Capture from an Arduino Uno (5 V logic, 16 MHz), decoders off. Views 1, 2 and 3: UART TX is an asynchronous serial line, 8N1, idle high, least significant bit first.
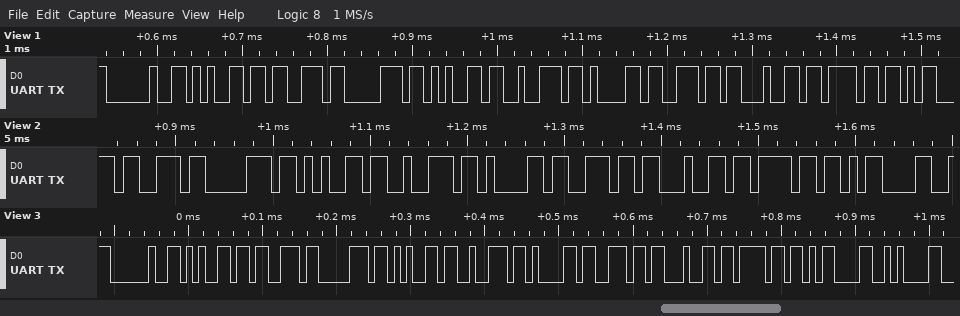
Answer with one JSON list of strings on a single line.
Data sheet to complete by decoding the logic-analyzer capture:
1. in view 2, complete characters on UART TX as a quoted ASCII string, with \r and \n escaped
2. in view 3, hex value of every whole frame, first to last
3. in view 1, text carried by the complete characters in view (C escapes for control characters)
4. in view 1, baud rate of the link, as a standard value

["\"sperando\\r\"", "20 65 73 70 65 72 61 6E 64 6F 0D 0A", "\" esperando\"", "115200 baud"]
